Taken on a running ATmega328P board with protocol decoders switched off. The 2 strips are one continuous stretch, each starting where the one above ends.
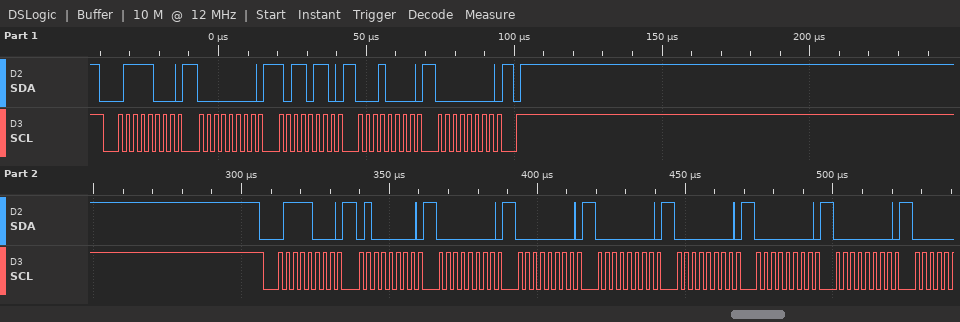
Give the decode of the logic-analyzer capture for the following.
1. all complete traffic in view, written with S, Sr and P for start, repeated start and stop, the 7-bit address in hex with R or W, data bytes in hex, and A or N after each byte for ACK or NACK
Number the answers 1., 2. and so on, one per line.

1. S 3CW A 00 A B6 A 10 A 00 A P S 3CW A 40 A 00 A 00 A 00 A 00 A 00 A 00 A
